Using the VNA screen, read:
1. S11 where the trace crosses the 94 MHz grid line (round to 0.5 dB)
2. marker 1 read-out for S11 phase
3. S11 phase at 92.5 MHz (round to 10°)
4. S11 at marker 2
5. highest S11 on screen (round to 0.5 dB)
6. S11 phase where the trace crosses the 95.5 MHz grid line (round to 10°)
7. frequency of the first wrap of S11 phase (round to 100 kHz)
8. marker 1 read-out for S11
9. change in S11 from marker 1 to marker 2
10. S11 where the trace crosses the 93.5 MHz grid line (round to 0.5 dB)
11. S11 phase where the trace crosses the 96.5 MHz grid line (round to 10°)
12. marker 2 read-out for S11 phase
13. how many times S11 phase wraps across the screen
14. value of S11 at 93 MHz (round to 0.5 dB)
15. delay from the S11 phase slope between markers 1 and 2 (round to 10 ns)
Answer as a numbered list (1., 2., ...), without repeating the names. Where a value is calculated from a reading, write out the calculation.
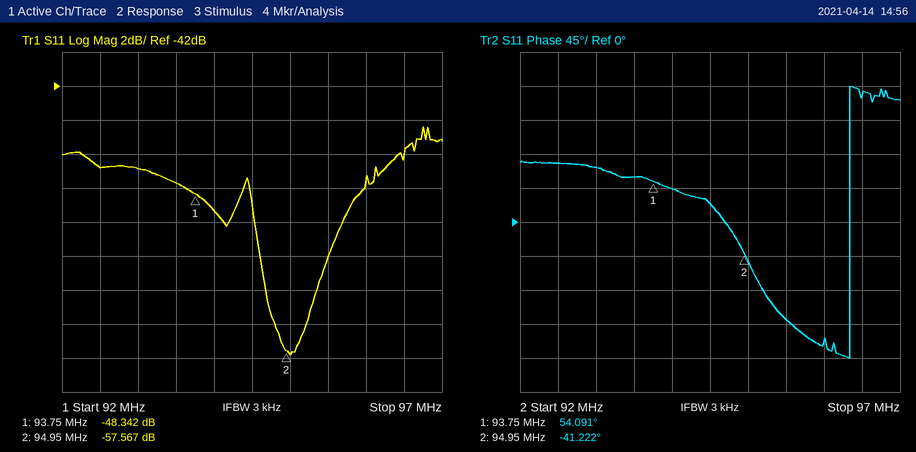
1. -49.5 dB
2. 54.091°
3. 80°
4. -57.567 dB
5. -44.5 dB
6. -130°
7. 96.3 MHz
8. -48.342 dB
9. -57.567 − (-48.342) = -9.225 dB
10. -47.5 dB
11. 170°
12. -41.222°
13. 1
14. -47.0 dB
15. −(-41.222° − (54.091°))/(360° × 1.2 MHz) ≈ 221 ns, so 220 ns to the nearest 10 ns
